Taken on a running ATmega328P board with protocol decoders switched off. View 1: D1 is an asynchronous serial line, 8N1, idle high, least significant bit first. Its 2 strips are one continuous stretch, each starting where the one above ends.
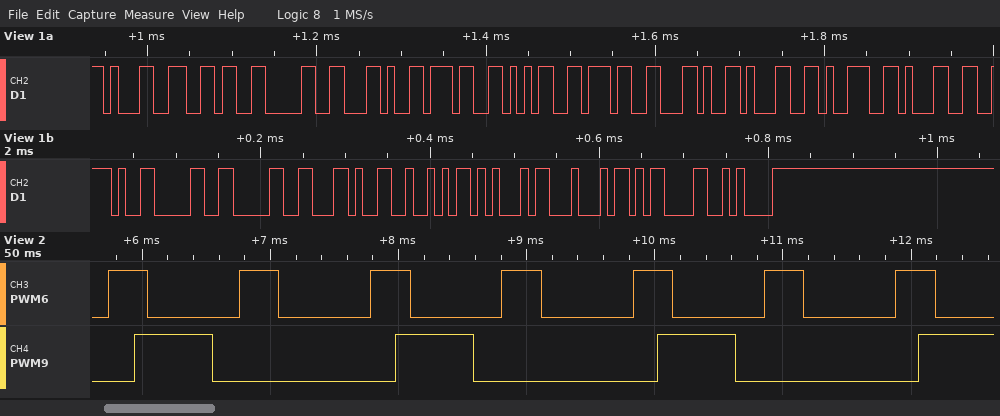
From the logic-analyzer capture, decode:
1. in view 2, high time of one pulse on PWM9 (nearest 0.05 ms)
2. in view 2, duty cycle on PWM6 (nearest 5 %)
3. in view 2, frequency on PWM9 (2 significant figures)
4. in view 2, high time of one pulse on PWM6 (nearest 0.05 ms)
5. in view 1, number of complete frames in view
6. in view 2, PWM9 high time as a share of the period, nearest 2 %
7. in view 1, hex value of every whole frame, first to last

0.60 ms
30 %
490 Hz
0.30 ms
20
30 %
31 36 30 2C 37 35 37 2C 31 39 31 2E 30 30 2C 52 45 44 0D 0A
